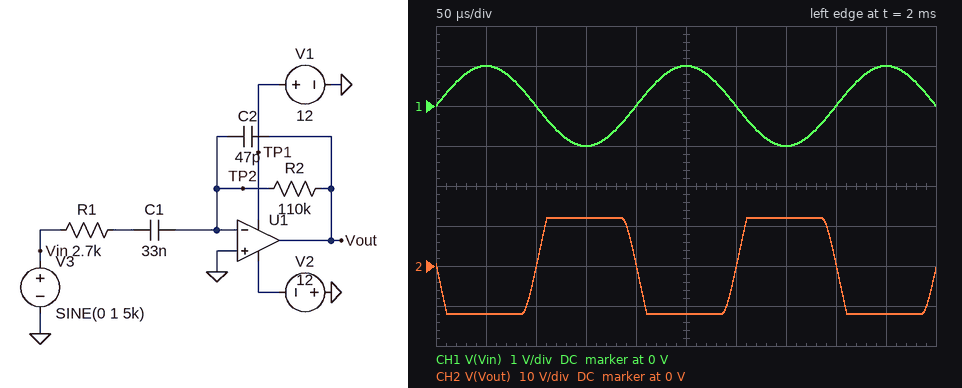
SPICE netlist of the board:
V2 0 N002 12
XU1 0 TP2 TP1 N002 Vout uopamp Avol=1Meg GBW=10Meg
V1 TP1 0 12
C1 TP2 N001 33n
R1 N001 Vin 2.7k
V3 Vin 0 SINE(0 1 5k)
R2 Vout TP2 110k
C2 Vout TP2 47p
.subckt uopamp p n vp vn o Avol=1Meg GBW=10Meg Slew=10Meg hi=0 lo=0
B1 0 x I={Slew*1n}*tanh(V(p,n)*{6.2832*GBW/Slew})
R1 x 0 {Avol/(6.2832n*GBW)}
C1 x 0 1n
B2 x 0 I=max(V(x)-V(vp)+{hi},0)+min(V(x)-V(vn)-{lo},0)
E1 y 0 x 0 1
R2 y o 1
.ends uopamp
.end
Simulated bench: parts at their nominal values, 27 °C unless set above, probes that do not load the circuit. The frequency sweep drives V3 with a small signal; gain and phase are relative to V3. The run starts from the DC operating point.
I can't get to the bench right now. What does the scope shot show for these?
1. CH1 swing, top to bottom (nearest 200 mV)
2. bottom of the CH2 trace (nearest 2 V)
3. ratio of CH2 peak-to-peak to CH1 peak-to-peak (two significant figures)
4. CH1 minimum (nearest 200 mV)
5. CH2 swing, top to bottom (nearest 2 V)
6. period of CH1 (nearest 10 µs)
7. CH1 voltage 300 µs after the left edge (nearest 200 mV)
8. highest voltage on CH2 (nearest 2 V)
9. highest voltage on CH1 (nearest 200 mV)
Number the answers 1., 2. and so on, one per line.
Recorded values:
1. 2.0 V
2. -12 V
3. 12
4. -1.0 V
5. 24 V
6. 200 µs
7. 0 V
8. 12 V
9. 1.0 V
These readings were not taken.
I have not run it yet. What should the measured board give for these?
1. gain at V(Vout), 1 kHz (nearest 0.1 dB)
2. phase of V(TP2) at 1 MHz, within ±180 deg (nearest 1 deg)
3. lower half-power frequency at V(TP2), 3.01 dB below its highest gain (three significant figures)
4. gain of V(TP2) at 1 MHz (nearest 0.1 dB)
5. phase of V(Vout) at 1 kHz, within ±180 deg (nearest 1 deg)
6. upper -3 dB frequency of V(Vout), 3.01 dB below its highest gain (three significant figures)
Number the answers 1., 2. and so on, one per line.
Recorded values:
1. 26.0 dB
2. -3 deg
3. 27.1 kHz
4. -19.1 dB
5. -121 deg
6. 30.5 kHz
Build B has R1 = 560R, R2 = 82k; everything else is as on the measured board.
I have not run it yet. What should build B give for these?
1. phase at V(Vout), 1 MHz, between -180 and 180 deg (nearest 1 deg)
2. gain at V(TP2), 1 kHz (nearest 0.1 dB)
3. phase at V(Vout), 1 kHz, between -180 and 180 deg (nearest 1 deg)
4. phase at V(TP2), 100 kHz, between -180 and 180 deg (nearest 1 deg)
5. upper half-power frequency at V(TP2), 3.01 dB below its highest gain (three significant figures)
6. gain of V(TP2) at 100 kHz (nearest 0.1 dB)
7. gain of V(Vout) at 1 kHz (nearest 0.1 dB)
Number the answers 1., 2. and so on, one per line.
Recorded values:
1. 88 deg
2. -55.4 dB
3. -98 deg
4. 17 deg
5. 16.1 MHz
6. -8.7 dB
7. 24.6 dB
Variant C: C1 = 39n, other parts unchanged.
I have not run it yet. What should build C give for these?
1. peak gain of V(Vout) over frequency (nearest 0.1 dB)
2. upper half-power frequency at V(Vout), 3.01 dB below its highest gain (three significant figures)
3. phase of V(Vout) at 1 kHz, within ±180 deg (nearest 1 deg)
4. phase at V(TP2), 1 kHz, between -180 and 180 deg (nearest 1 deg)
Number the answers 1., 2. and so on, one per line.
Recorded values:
1. 31.8 dB
2. 30.1 kHz
3. -125 deg
4. 144 deg
